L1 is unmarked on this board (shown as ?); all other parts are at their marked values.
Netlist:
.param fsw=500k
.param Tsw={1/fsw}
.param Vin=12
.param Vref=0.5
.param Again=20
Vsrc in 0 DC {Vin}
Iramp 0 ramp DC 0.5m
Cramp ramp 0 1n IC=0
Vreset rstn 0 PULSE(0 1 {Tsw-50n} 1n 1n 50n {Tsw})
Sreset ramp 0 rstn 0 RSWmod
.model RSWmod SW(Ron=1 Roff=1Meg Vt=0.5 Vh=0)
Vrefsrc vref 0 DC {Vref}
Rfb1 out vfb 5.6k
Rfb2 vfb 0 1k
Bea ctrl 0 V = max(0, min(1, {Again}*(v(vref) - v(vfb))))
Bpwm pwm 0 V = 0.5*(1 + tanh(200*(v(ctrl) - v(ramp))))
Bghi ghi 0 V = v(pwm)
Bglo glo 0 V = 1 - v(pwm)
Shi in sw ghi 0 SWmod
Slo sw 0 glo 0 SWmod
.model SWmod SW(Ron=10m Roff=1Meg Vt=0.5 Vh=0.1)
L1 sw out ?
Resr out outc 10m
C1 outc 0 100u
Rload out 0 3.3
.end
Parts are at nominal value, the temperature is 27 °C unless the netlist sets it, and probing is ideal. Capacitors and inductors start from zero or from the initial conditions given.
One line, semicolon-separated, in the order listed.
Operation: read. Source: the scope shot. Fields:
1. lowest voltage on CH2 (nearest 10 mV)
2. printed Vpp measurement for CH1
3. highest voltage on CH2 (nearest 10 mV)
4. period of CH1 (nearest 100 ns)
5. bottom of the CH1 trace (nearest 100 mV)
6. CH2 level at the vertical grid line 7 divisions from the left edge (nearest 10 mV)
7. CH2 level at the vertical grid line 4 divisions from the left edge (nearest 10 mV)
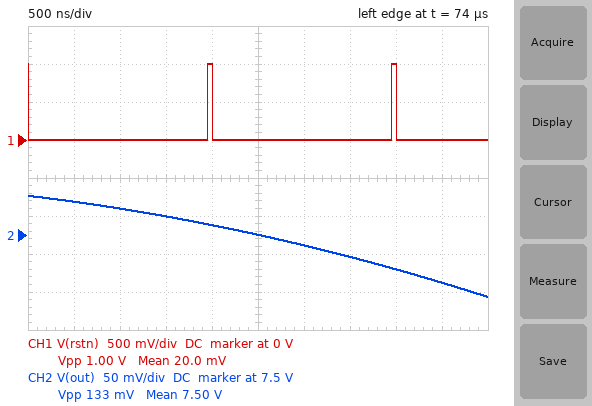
7.42 V; 1.00 V; 7.55 V; 2.0 µs; 0 V; 7.47 V; 7.51 V
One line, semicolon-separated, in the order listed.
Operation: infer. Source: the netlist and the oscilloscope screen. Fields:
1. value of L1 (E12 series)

15 µH
